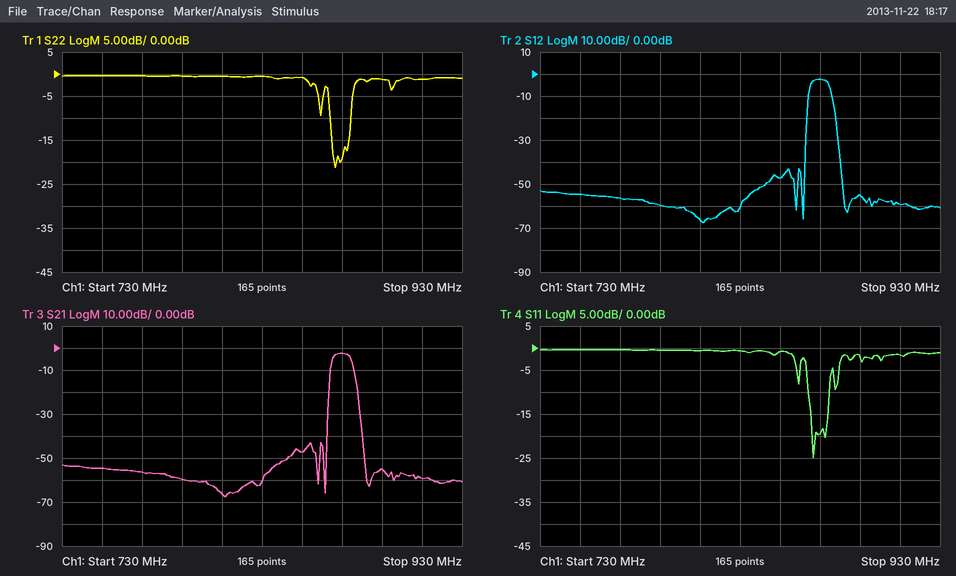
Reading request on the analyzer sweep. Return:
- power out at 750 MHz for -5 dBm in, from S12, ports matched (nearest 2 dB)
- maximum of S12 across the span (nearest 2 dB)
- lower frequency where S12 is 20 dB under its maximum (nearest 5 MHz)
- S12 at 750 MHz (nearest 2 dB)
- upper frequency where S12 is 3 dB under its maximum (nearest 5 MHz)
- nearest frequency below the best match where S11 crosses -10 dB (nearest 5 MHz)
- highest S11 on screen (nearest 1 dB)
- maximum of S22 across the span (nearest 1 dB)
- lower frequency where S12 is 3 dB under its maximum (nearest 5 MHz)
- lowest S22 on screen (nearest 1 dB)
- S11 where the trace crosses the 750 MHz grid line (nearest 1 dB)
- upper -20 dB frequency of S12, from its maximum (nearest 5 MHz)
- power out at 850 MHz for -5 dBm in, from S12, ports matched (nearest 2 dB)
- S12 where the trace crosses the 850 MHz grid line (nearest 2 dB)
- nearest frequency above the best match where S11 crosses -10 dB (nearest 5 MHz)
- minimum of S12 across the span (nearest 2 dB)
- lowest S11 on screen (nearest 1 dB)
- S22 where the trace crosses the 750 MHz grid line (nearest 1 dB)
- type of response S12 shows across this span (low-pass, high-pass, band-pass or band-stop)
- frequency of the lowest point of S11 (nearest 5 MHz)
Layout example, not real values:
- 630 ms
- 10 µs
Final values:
- -60 dBm
- -2 dB
- 865 MHz
- -54 dB
- 875 MHz
- 865 MHz
- 0 dB
- 0 dB
- 865 MHz
- -21 dB
- 0 dB
- 880 MHz
- -52 dBm
- -48 dB
- 875 MHz
- -68 dB
- -25 dB
- 0 dB
- band-pass
- 865 MHz
